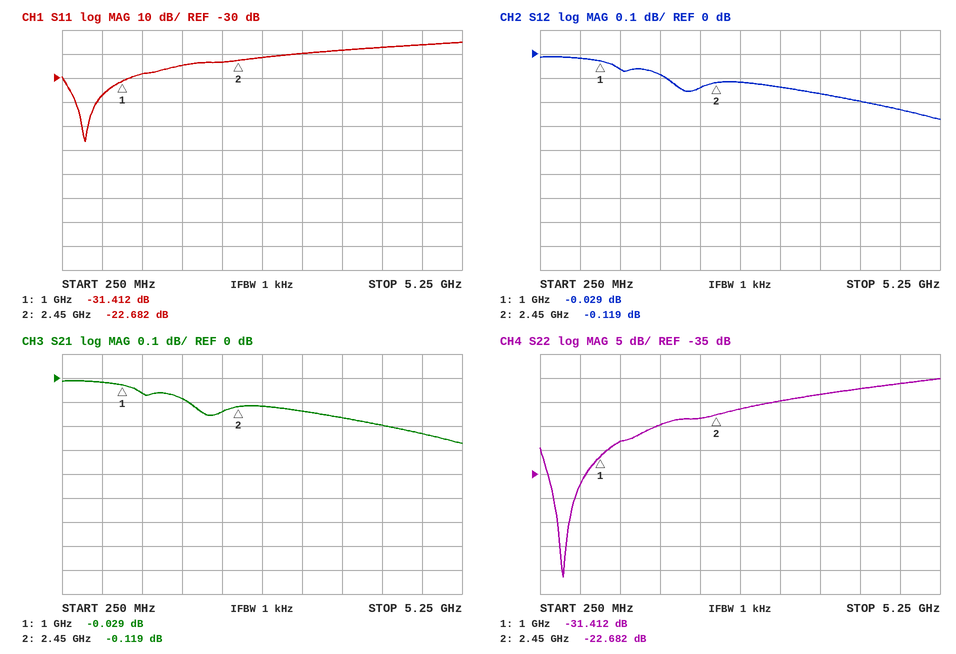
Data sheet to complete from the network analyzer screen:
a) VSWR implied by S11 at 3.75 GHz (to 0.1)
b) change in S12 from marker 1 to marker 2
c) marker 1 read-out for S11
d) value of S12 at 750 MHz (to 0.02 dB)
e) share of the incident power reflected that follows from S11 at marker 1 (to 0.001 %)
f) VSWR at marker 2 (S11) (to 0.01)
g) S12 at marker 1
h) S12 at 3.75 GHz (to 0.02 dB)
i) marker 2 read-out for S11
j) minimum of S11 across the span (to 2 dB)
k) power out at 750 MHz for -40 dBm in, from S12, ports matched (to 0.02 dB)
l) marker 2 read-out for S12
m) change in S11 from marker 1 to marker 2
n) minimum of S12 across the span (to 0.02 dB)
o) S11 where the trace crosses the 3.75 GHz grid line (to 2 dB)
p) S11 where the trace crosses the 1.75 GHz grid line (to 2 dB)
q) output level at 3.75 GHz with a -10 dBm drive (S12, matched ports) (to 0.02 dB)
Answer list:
1.3
-0.090 dB
-31.412 dB
-0.02 dB
0.072 %
1.16
-0.029 dB
-0.16 dB
-22.682 dB
-56 dB
-40.02 dBm
-0.119 dB
8.730 dB
-0.28 dB
-18 dB
-24 dB
-10.16 dBm
